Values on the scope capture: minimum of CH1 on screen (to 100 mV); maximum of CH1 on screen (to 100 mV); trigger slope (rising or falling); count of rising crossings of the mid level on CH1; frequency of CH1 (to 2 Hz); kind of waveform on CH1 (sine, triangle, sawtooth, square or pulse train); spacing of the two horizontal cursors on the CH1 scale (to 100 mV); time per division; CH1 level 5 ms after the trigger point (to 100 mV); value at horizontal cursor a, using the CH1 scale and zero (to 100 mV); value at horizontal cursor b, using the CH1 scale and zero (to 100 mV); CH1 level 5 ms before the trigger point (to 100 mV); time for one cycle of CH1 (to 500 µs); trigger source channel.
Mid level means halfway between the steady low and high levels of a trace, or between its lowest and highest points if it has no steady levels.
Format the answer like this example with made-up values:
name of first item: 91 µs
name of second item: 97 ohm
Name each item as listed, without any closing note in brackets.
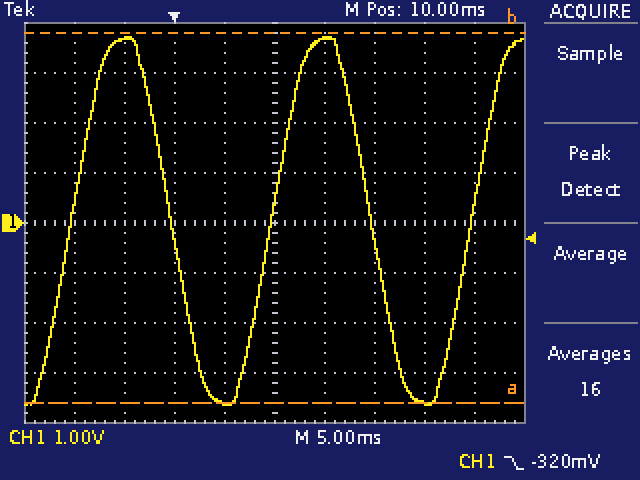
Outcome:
minimum of CH1 on screen: -3.6 V
maximum of CH1 on screen: 3.7 V
trigger slope: falling
count of rising crossings of the mid level on CH1: 3
frequency of CH1: 50 Hz
kind of waveform on CH1: sine
spacing of the two horizontal cursors on the CH1 scale: 7.4 V
time per division: 5 ms
CH1 level 5 ms after the trigger point: -3.6 V
value at horizontal cursor a, using the CH1 scale and zero: -3.6 V
value at horizontal cursor b, using the CH1 scale and zero: 3.8 V
CH1 level 5 ms before the trigger point: 3.7 V
time for one cycle of CH1: 20.0 ms
trigger source channel: CH1
